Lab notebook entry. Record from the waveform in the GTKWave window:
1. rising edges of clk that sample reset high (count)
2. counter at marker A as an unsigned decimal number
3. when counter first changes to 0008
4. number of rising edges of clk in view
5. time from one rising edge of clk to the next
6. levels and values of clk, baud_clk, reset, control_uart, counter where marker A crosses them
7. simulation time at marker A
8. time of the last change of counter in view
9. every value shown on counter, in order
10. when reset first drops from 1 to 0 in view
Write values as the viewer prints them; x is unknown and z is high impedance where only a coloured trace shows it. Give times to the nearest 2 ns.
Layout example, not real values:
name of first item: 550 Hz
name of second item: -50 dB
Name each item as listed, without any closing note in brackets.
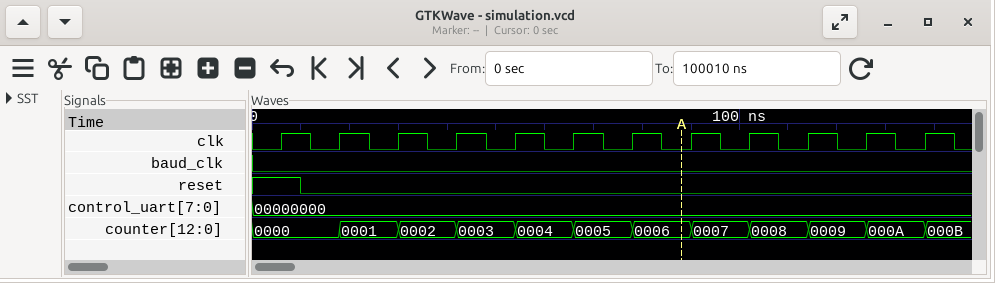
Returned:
rising edges of clk that sample reset high: 1
counter at marker A as an unsigned decimal number: 6
when counter first changes to 0008: 102 ns
number of rising edges of clk in view: 12
time from one rising edge of clk to the next: 12 ns
levels and values of clk, baud_clk, reset, control_uart, counter where marker A crosses them: clk=0, baud_clk=0, reset=0, control_uart=00000000, counter=0006
simulation time at marker A: 88 ns
time of the last change of counter in view: 138 ns
every value shown on counter, in order: 0000, 0001, 0002, 0003, 0004, 0005, 0006, 0007, 0008, 0009, 000A, 000B
when reset first drops from 1 to 0 in view: 10 ns
